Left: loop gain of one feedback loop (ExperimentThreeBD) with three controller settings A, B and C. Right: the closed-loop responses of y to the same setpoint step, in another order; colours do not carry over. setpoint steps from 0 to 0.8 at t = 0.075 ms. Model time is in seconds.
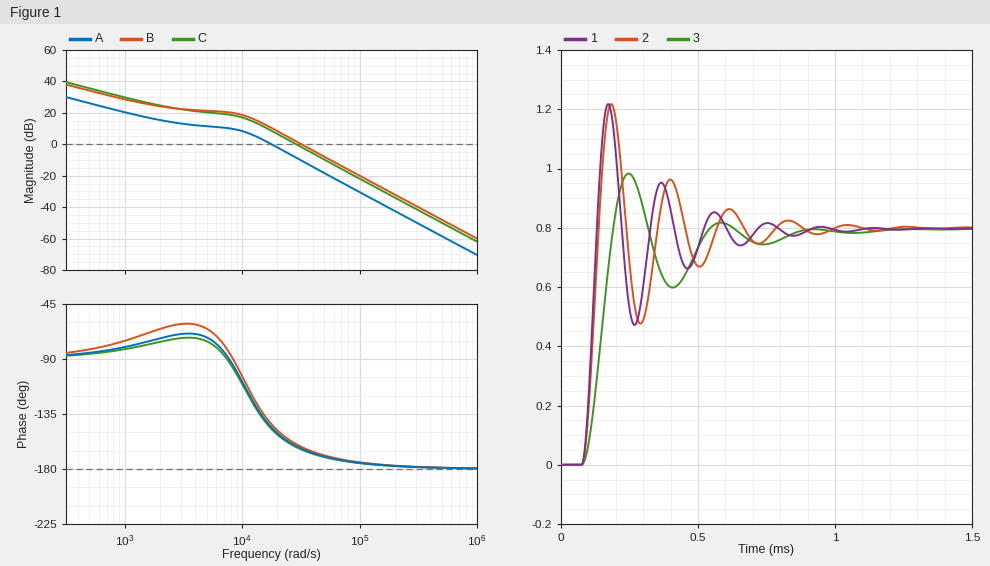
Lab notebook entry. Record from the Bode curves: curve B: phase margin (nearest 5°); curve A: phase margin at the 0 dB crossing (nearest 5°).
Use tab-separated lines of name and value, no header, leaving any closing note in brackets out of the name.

curve B: phase margin	20°
curve A: phase margin at the 0 dB crossing	35°
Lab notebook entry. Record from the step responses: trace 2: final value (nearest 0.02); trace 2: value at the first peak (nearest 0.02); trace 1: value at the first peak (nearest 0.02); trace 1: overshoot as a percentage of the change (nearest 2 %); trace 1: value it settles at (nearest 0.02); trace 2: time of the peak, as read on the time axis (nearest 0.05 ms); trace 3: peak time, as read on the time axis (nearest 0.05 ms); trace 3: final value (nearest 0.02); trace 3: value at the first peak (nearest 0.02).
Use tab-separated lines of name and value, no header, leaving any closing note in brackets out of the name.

trace 2: final value	0.80
trace 2: value at the first peak	1.22
trace 1: value at the first peak	1.22
trace 1: overshoot as a percentage of the change	52 %
trace 1: value it settles at	0.80
trace 2: time of the peak, as read on the time axis	0.20 ms
trace 3: peak time, as read on the time axis	0.25 ms
trace 3: final value	0.80
trace 3: value at the first peak	0.98
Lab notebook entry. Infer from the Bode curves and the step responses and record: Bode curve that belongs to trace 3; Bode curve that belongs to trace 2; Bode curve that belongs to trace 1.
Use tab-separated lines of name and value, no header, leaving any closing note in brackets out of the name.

Bode curve that belongs to trace 3	A
Bode curve that belongs to trace 2	C
Bode curve that belongs to trace 1	B
